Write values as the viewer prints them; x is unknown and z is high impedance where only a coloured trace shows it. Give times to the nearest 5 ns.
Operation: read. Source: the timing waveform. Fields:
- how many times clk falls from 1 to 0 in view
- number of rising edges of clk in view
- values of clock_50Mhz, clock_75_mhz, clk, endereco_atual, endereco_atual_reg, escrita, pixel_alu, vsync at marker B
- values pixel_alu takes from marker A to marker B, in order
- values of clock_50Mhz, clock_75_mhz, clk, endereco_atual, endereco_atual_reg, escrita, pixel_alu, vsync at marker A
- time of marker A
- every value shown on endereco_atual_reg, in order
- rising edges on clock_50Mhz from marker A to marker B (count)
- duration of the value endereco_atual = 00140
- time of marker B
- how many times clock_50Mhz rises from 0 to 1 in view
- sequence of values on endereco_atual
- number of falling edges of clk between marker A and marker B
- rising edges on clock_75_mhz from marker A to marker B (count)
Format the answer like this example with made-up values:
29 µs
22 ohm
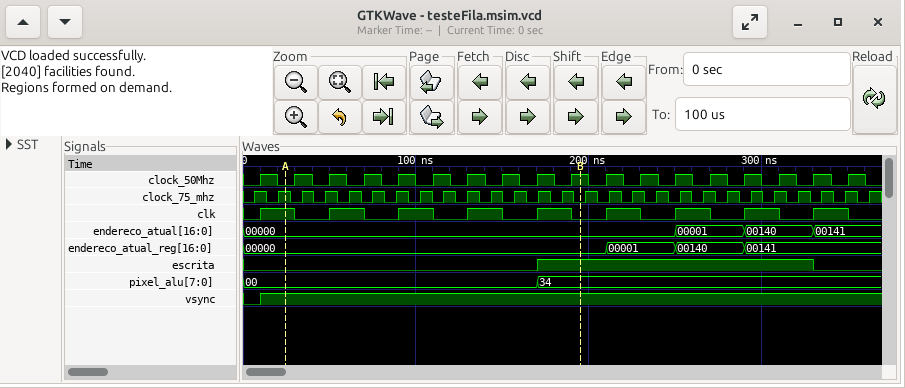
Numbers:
9
9
clock_50Mhz=1, clock_75_mhz=0, clk=0, endereco_atual=00000, endereco_atual_reg=00000, escrita=1, pixel_alu=34, vsync=1
00, 34
clock_50Mhz=0, clock_75_mhz=1, clk=1, endereco_atual=00000, endereco_atual_reg=00000, escrita=0, pixel_alu=00, vsync=1
25 ns
00000, 00001, 00140, 00141
9
40 ns
195 ns
18
00000, 00001, 00140, 00141
5
12
